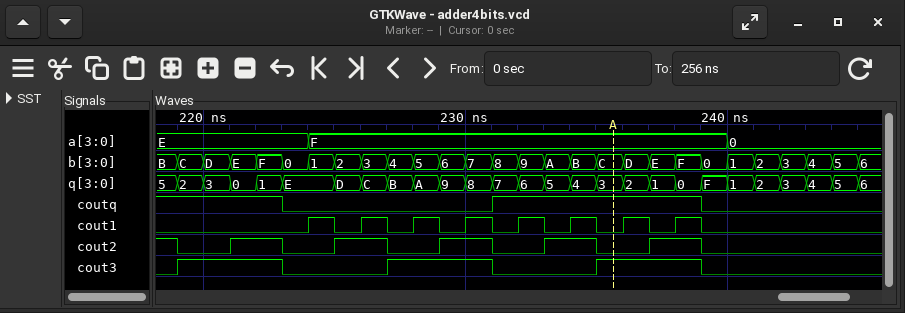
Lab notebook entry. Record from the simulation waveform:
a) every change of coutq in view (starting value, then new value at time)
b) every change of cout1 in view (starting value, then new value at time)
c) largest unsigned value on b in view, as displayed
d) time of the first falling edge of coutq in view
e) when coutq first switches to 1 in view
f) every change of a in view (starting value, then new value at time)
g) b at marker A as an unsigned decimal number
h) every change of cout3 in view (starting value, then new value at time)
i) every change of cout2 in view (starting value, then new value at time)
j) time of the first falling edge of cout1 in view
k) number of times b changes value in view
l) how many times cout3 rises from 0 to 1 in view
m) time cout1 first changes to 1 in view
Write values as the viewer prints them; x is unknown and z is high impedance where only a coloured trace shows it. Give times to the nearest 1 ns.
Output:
1, 0 at 223 ns, 1 at 231 ns, 0 at 239 ns
0, 1 at 224 ns, 0 at 225 ns, 1 at 226 ns, 0 at 227 ns, 1 at 228 ns, 0 at 229 ns, 1 at 230 ns, 0 at 231 ns, 1 at 232 ns, 0 at 233 ns, 1 at 234 ns, 0 at 235 ns, 1 at 236 ns, 0 at 237 ns, 1 at 238 ns, 0 at 239 ns
F
223 ns
231 ns
E, F at 224 ns, 0 at 240 ns
12
0, 1 at 219 ns, 0 at 223 ns, 1 at 227 ns, 0 at 231 ns, 1 at 235 ns, 0 at 239 ns
1, 0 at 219 ns, 1 at 221 ns, 0 at 223 ns, 1 at 225 ns, 0 at 227 ns, 1 at 229 ns, 0 at 231 ns, 1 at 233 ns, 0 at 235 ns, 1 at 237 ns, 0 at 239 ns
225 ns
27
3
224 ns
